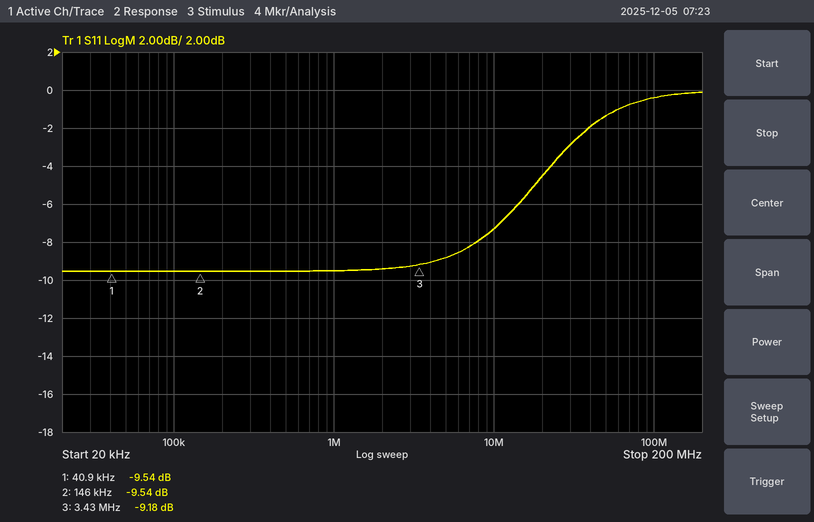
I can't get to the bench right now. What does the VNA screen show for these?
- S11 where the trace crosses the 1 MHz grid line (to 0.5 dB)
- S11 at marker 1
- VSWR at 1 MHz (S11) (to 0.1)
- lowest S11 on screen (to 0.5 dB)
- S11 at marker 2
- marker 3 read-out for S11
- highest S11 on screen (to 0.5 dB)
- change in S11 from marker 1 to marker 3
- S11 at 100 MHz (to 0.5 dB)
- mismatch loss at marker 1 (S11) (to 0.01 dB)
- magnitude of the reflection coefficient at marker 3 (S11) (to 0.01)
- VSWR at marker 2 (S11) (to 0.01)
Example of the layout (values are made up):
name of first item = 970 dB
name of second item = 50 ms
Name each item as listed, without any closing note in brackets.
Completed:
S11 where the trace crosses the 1 MHz grid line = -9.5 dB
S11 at marker 1 = -9.54 dB
VSWR at 1 MHz (S11) = 2.0
lowest S11 on screen = -9.5 dB
S11 at marker 2 = -9.54 dB
marker 3 read-out for S11 = -9.18 dB
highest S11 on screen = 0.0 dB
change in S11 from marker 1 to marker 3 = 0.36 dB
S11 at 100 MHz = -0.5 dB
mismatch loss at marker 1 (S11) = 0.51 dB
magnitude of the reflection coefficient at marker 3 (S11) = 0.35
VSWR at marker 2 (S11) = 2.00
